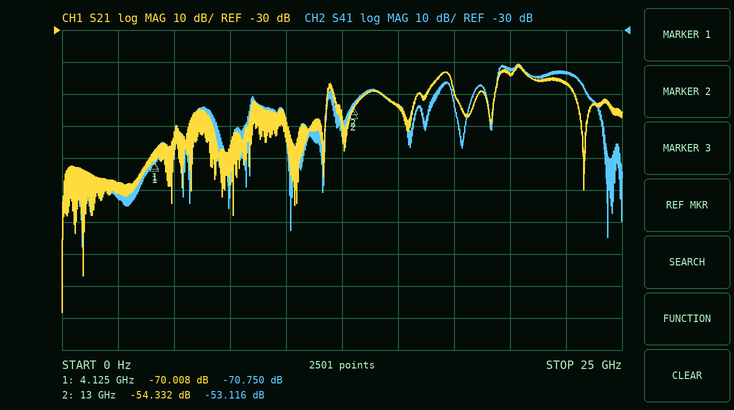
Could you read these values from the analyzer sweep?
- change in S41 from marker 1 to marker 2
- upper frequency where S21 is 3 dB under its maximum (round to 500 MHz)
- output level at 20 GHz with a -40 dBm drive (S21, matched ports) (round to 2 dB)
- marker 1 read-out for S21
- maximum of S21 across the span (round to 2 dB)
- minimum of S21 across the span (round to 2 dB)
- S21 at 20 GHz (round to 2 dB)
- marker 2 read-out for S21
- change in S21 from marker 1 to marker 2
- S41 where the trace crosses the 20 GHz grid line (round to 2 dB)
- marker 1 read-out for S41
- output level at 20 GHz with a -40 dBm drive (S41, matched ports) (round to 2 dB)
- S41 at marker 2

17.634 dB
20.5 GHz
-84 dBm
-70.008 dB
-40 dB
-118 dB
-44 dB
-54.332 dB
15.676 dB
-42 dB
-70.750 dB
-82 dBm
-53.116 dB
